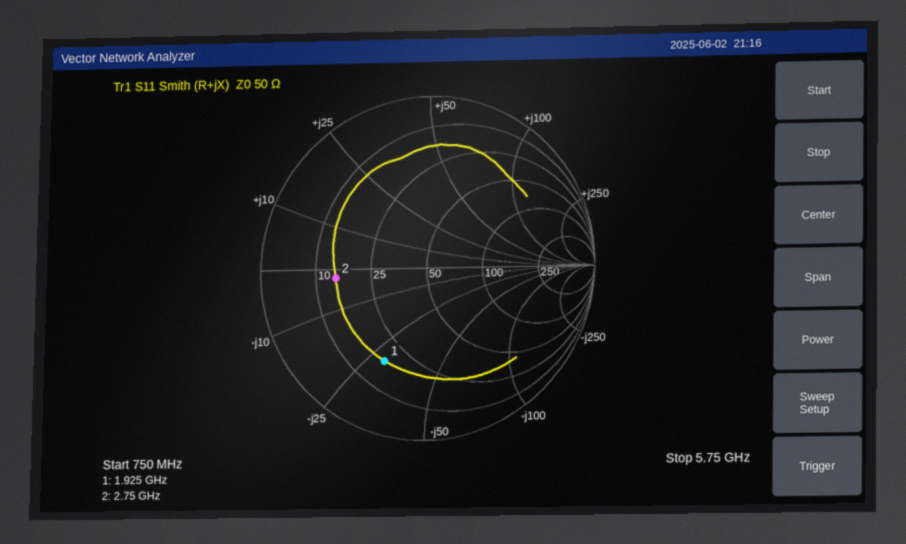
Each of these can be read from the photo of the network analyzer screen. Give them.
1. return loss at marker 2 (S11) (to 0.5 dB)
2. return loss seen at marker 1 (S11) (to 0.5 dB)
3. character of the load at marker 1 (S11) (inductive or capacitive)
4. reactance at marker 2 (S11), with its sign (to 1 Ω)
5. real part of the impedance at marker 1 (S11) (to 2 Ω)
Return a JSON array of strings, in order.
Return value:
["5.0 dB", "4.5 dB", "capacitive", "-2 Ω", "18 Ω"]
